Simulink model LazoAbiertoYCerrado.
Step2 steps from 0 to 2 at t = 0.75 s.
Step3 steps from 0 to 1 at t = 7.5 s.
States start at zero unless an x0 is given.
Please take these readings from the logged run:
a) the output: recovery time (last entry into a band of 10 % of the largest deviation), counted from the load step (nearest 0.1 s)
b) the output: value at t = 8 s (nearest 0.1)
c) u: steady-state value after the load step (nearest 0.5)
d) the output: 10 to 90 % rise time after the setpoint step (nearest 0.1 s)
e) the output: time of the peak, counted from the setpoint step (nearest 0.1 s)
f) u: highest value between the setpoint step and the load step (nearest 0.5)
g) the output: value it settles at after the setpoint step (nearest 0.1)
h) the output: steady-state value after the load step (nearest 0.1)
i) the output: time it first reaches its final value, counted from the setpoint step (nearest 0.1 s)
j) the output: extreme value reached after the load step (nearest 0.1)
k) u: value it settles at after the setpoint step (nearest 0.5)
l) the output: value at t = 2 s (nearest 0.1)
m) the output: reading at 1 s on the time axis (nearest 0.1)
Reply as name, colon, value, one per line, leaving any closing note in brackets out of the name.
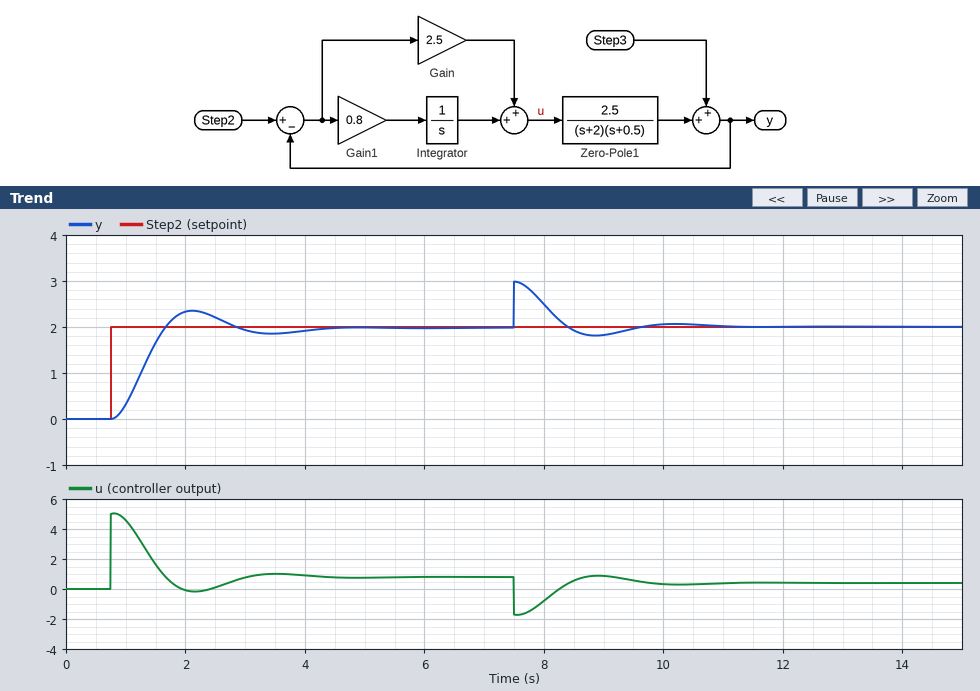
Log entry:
the output: recovery time (last entry into a band of 10 % of the largest deviation), counted from the load step: 1.8 s
the output: value at t = 8 s: 2.5
u: steady-state value after the load step: 0.5
the output: 10 to 90 % rise time after the setpoint step: 0.6 s
the output: time of the peak, counted from the setpoint step: 1.4 s
u: highest value between the setpoint step and the load step: 5.0
the output: value it settles at after the setpoint step: 2.0
the output: steady-state value after the load step: 2.0
the output: time it first reaches its final value, counted from the setpoint step: 0.9 s
the output: extreme value reached after the load step: 3.0
u: value it settles at after the setpoint step: 1.0
the output: value at t = 2 s: 2.3
the output: reading at 1 s on the time axis: 0.3
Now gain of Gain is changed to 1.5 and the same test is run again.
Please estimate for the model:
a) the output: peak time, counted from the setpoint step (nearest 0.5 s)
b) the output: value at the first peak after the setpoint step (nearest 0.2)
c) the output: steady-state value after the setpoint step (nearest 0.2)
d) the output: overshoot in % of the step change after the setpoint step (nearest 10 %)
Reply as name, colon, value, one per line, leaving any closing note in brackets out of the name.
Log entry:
the output: peak time, counted from the setpoint step: 2.0 s
the output: value at the first peak after the setpoint step: 2.4
the output: steady-state value after the setpoint step: 2.0
the output: overshoot in % of the step change after the setpoint step: 20 %
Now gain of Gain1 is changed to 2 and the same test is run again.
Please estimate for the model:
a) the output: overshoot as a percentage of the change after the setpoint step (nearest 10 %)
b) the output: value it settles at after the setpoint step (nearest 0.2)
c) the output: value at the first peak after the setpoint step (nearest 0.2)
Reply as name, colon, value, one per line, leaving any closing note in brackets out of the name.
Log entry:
the output: overshoot as a percentage of the change after the setpoint step: 40 %
the output: value it settles at after the setpoint step: 2.0
the output: value at the first peak after the setpoint step: 2.8
